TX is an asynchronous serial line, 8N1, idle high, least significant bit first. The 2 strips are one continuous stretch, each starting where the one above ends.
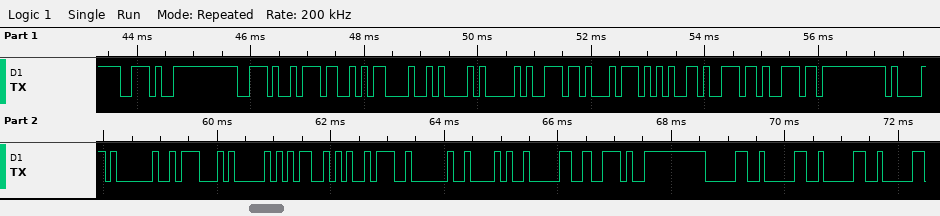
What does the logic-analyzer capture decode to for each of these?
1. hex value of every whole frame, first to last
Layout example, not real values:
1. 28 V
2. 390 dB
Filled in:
1. 0x2E 0x2E 0x37 0x0D 0x0A 0x41 0x6E 0x74 0x65 0x6E 0x6E 0x61 0x20 0x47 0x50 0x53 0x3A 0x20 0x28 0x30 0x2E 0x30 0x30 0x30
